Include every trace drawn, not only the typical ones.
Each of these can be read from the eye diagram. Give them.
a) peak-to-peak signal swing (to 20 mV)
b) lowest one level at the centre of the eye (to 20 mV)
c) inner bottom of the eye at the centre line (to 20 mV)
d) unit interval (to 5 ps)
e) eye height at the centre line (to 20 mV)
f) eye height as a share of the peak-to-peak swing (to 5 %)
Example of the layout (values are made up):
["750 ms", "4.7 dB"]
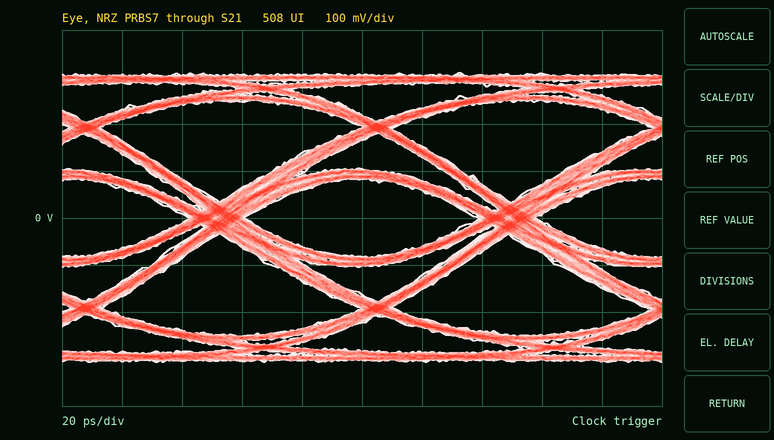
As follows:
["620 mV", "80 mV", "-80 mV", "95 ps", "160 mV", "25 %"]
